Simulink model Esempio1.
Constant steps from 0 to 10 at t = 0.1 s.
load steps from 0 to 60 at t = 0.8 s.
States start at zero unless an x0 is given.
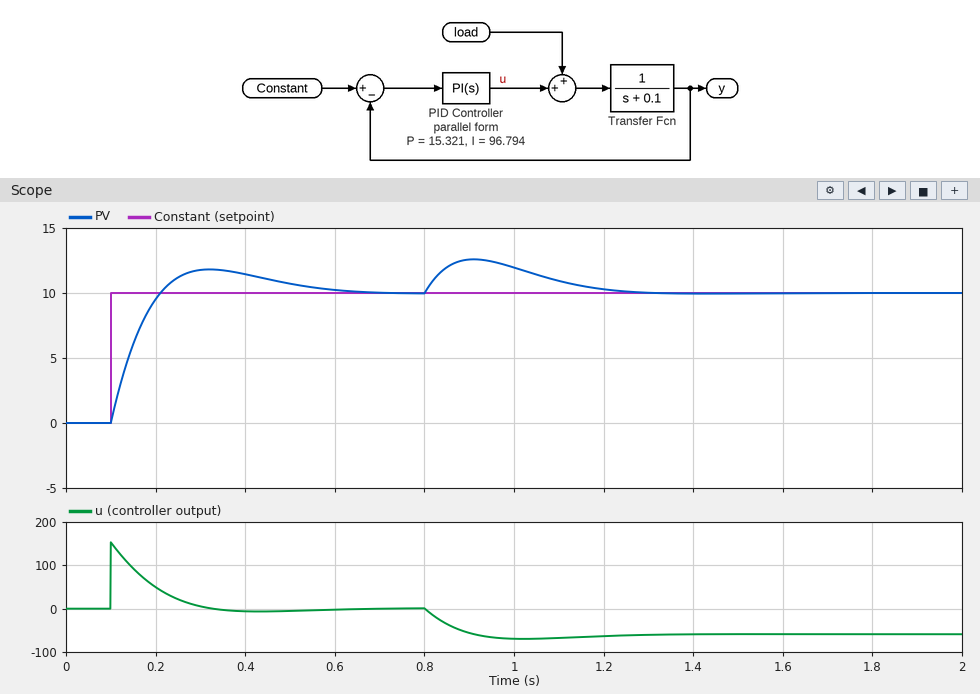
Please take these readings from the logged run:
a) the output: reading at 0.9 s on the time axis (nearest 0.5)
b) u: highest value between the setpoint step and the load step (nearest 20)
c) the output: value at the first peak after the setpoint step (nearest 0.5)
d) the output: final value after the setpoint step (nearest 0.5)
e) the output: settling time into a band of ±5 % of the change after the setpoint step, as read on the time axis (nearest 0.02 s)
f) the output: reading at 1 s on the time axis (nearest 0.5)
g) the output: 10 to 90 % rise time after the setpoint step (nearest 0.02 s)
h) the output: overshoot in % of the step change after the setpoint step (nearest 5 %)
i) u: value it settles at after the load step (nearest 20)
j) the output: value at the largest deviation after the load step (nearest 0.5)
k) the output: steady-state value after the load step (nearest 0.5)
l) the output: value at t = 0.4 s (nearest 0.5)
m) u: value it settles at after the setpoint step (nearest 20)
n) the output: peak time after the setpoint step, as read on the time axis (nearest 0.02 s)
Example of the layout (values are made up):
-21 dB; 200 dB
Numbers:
12.5; 160; 12.0; 10.0; 0.54 s; 12.0; 0.08 s; 20 %; -60; 12.5; 10.0; 11.5; 0; 0.32 s
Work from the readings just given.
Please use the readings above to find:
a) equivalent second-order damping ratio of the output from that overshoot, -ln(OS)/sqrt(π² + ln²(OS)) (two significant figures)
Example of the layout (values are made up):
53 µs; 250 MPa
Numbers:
0.46
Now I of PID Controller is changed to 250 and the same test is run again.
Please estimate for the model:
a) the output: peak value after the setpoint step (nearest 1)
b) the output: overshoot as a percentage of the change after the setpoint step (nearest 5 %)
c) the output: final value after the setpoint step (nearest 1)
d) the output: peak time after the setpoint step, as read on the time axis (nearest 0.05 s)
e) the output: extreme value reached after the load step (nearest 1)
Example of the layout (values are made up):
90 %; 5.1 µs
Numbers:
13; 30 %; 10; 0.25 s; 12
